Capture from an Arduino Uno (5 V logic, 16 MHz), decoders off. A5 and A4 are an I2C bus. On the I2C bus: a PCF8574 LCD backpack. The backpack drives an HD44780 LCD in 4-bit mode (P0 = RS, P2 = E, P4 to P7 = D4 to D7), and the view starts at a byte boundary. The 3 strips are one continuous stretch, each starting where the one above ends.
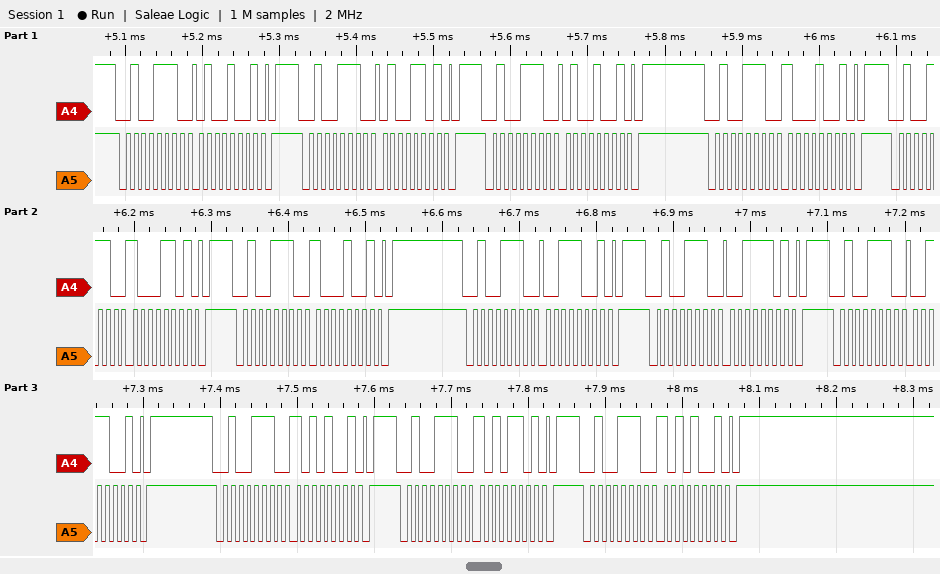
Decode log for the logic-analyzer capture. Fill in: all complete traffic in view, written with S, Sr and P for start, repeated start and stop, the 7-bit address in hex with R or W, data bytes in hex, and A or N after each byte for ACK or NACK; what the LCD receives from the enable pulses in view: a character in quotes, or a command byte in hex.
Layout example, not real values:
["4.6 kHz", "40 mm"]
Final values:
["S 27W A 49 A P S 27W A 4D A P S 27W A 49 A P S 27W A 89 A P S 27W A 8D A P S 27W A 89 A P S 27W A 39 A P S 27W A 3D A P S 27W A 39 A P S 27W A A9 A P S 27W A AD A P S 27W A A9 A P", "'H' ':'"]
